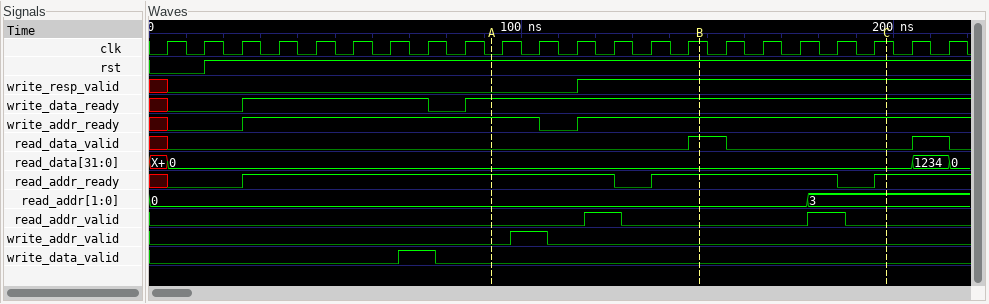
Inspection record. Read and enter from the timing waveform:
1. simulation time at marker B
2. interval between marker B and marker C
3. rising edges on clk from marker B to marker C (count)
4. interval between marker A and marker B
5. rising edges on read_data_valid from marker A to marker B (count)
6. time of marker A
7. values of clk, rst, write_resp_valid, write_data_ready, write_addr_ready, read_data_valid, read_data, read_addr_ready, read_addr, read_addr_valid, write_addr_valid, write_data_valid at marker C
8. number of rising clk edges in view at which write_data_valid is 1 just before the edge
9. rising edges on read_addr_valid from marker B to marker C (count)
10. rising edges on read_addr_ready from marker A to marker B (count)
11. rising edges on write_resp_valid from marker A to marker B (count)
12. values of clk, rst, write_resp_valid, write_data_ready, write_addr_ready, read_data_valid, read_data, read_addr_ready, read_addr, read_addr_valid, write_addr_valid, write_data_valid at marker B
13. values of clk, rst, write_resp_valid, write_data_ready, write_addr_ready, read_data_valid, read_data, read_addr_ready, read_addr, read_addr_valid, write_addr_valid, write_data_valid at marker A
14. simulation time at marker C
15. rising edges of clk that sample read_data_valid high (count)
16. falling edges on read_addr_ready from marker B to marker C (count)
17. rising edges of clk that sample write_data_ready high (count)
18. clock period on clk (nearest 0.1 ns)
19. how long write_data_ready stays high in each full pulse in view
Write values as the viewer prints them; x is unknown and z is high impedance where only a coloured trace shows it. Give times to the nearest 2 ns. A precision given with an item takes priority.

148 ns
50 ns
5
56 ns
1
92 ns
clk=1, rst=1, write_resp_valid=1, write_data_ready=1, write_addr_ready=1, read_data_valid=0, read_data=0, read_addr_ready=1, read_addr=3, read_addr_valid=0, write_addr_valid=0, write_data_valid=0
1
1
1
1
clk=1, rst=1, write_resp_valid=1, write_data_ready=1, write_addr_ready=1, read_data_valid=1, read_data=0, read_addr_ready=1, read_addr=0, read_addr_valid=0, write_addr_valid=0, write_data_valid=0
clk=0, rst=1, write_resp_valid=0, write_data_ready=1, write_addr_ready=1, read_data_valid=0, read_data=0, read_addr_ready=1, read_addr=0, read_addr_valid=0, write_addr_valid=0, write_data_valid=0
198 ns
2
1
18
10 ns
50 ns
